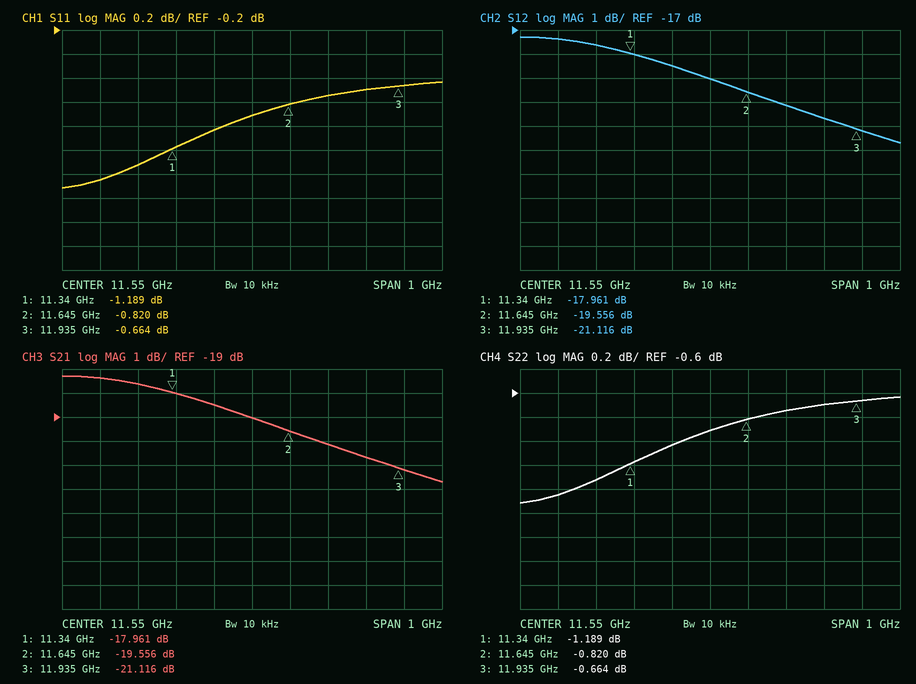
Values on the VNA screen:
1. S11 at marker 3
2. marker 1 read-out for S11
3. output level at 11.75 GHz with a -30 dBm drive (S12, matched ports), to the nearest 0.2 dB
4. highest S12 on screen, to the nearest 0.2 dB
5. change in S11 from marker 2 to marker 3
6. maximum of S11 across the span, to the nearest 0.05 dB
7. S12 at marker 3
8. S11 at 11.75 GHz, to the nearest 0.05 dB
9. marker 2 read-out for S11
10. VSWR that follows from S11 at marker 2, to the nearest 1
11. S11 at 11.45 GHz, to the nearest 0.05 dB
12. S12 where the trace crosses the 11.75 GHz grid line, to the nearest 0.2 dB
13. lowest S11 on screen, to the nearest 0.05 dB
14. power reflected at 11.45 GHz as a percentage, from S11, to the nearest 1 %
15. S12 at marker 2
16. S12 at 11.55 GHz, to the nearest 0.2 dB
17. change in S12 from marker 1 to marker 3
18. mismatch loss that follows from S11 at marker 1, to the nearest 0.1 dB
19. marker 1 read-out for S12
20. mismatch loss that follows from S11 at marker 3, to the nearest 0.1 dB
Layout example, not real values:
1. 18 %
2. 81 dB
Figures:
1. -0.664 dB
2. -1.189 dB
3. -50.2 dBm
4. -17.2 dB
5. 0.156 dB
6. -0.65 dB
7. -21.116 dB
8. -0.75 dB
9. -0.820 dB
10. 21
11. -1.05 dB
12. -20.2 dB
13. -1.50 dB
14. 79 %
15. -19.556 dB
16. -19.0 dB
17. -3.155 dB
18. 6.2 dB
19. -17.961 dB
20. 8.5 dB
